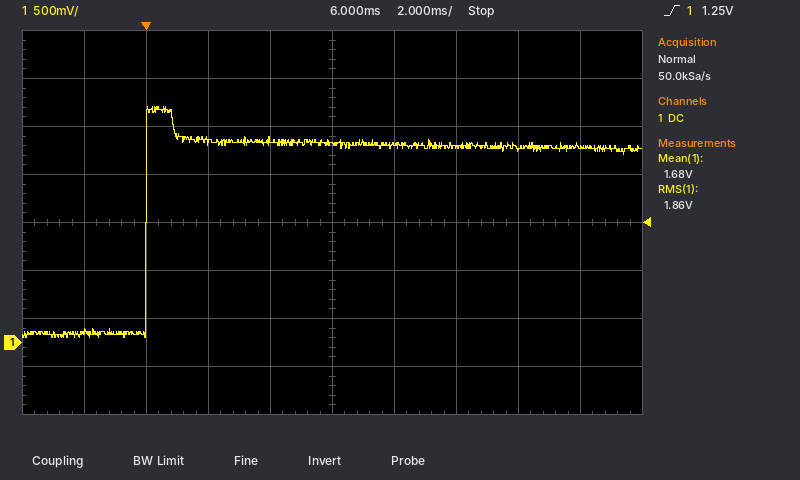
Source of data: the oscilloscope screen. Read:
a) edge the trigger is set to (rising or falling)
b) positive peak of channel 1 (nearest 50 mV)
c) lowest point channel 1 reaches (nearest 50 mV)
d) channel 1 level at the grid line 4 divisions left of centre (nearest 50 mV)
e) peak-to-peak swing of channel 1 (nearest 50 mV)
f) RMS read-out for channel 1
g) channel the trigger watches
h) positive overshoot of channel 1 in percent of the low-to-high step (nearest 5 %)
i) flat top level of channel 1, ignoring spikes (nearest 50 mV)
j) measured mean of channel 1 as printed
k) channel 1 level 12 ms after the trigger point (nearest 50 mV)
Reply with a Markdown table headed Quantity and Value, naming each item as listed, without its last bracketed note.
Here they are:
| Quantity | Value |
|---|---|
| edge the trigger is set to | rising |
| positive peak of channel 1 | 2.45 V |
| lowest point channel 1 reaches | 50 mV |
| channel 1 level at the grid line 4 divisions left of centre | 100 mV |
| peak-to-peak swing of channel 1 | 2.40 V |
| RMS read-out for channel 1 | 1.86 V |
| channel the trigger watches | channel 1 |
| positive overshoot of channel 1 in percent of the low-to-high step | 20 % |
| flat top level of channel 1, ignoring spikes | 2.05 V |
| measured mean of channel 1 as printed | 1.68 V |
| channel 1 level 12 ms after the trigger point | 2.00 V |
